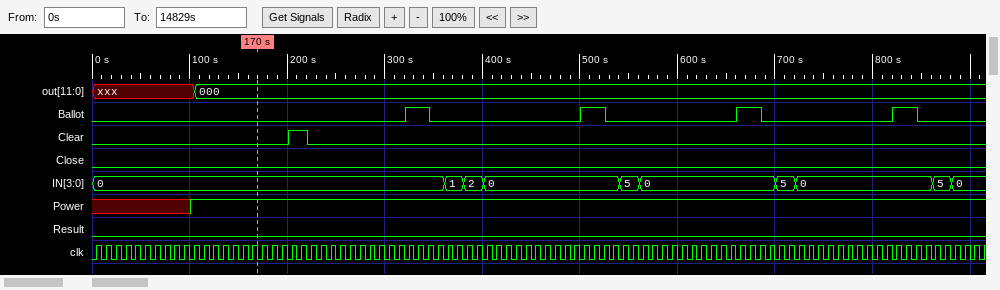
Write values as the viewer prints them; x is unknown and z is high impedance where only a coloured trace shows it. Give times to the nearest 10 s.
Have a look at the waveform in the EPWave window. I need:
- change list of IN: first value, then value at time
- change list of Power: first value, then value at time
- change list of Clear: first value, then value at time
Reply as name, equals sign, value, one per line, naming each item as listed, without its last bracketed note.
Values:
change list of IN: first value, then value at time = 0, 1 at 360 s, 2 at 380 s, 0 at 400 s, 5 at 540 s, 0 at 560 s, 5 at 700 s, 0 at 720 s, 5 at 860 s, 0 at 880 s
change list of Power: first value, then value at time = x, 1 at 100 s
change list of Clear: first value, then value at time = 0, 1 at 200 s, 0 at 220 s
